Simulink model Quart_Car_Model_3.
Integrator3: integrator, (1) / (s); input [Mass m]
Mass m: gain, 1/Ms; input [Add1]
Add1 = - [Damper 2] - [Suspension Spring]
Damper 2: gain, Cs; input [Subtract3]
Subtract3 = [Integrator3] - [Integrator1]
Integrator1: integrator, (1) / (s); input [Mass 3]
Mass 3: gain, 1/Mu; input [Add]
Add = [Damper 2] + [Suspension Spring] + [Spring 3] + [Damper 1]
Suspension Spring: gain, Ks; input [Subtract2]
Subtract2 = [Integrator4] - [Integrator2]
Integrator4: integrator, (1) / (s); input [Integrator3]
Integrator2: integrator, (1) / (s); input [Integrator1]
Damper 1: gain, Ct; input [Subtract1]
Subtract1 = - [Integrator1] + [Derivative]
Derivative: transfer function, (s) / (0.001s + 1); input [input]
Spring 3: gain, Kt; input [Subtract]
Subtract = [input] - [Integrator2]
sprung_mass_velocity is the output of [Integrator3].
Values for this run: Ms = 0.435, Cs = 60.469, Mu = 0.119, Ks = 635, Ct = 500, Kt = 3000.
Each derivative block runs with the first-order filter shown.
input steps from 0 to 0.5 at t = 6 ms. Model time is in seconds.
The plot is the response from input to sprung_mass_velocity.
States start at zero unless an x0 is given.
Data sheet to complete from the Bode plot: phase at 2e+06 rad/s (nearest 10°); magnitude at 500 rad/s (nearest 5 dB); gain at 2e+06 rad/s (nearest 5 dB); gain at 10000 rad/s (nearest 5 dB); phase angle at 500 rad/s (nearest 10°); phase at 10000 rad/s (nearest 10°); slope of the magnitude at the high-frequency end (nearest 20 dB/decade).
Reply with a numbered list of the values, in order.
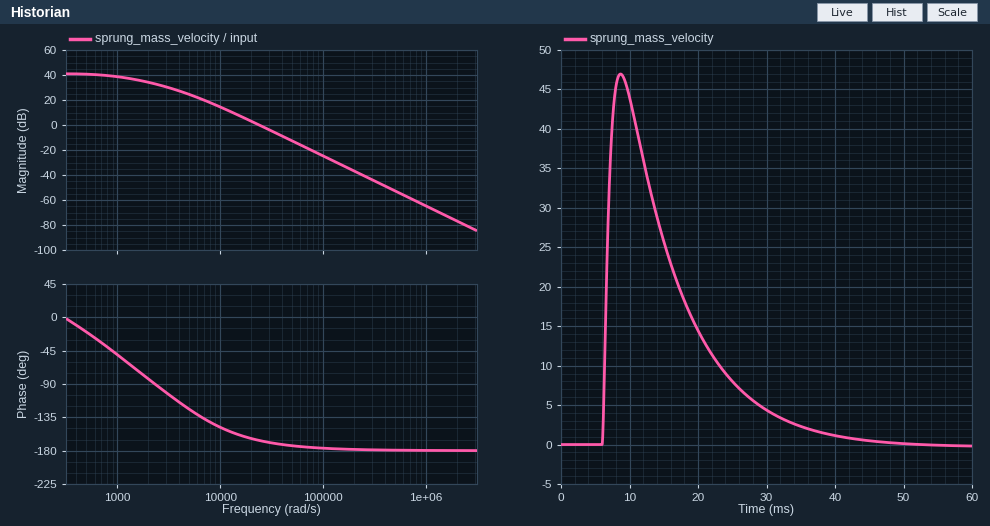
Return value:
1. -180°
2. 40 dB
3. -75 dB
4. 15 dB
5. -20°
6. -150°
7. -40 dB/decade
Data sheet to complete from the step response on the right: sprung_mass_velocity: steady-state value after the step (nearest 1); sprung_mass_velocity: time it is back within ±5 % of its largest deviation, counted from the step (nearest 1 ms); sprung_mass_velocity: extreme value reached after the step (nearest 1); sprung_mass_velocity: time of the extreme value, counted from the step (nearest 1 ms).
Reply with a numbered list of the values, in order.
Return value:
1. 0
2. 29 ms
3. 47
4. 3 ms
